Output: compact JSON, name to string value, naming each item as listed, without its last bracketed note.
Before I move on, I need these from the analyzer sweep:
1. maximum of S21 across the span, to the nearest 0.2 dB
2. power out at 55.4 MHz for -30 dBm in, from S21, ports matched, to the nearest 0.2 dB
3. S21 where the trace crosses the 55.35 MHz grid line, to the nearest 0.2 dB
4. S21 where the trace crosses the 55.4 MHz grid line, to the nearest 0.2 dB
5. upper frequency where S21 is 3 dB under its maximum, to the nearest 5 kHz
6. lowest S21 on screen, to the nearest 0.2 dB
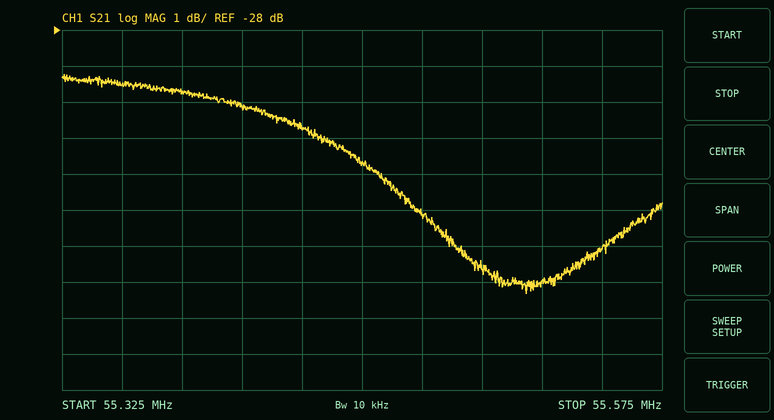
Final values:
{"maximum of S21 across the span, to the nearest 0.2 dB": "-29.2 dB", "power out at 55.4 MHz for -30 dBm in, from S21, ports matched, to the nearest 0.2 dB": "-60.2 dBm", "S21 where the trace crosses the 55.35 MHz grid line, to the nearest 0.2 dB": "-29.6 dB", "S21 where the trace crosses the 55.4 MHz grid line, to the nearest 0.2 dB": "-30.2 dB", "upper frequency where S21 is 3 dB under its maximum, to the nearest 5 kHz": "55.460 MHz", "lowest S21 on screen, to the nearest 0.2 dB": "-35.4 dB"}
